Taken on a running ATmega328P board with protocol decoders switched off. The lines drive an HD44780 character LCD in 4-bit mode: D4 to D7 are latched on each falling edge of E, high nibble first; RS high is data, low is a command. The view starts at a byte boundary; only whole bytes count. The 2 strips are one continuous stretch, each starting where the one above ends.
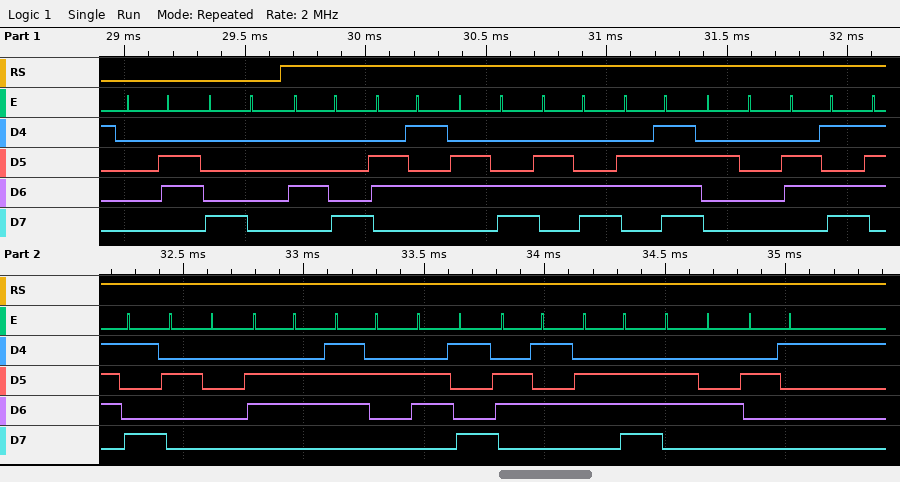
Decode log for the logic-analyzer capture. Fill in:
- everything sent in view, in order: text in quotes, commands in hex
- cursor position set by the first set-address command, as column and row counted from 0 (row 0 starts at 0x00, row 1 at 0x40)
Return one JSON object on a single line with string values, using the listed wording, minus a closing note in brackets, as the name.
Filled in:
{"everything sent in view, in order: text in quotes, commands in hex": "0x06 0x80 \"Hello my friend!\"", "cursor position set by the first set-address command, as column and row counted from 0": "column 0, row 0"}
